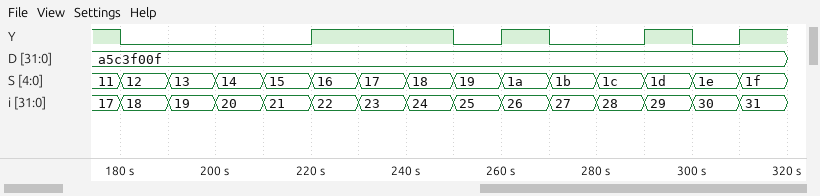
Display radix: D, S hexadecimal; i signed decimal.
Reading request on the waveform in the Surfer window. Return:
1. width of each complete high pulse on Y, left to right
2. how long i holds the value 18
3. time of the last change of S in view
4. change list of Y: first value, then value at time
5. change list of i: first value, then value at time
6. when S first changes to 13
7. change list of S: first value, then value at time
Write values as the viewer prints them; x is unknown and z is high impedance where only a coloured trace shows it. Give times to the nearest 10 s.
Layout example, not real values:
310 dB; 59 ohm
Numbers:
30 s, 10 s, 10 s; 10 s; 310 s; 1, 0 at 180 s, 1 at 220 s, 0 at 250 s, 1 at 260 s, 0 at 270 s, 1 at 290 s, 0 at 300 s, 1 at 310 s; 17, 18 at 180 s, 19 at 190 s, 20 at 200 s, 21 at 210 s, 22 at 220 s, 23 at 230 s, 24 at 240 s, 25 at 250 s, 26 at 260 s, 27 at 270 s, 28 at 280 s, 29 at 290 s, 30 at 300 s, 31 at 310 s; 190 s; 11, 12 at 180 s, 13 at 190 s, 14 at 200 s, 15 at 210 s, 16 at 220 s, 17 at 230 s, 18 at 240 s, 19 at 250 s, 1a at 260 s, 1b at 270 s, 1c at 280 s, 1d at 290 s, 1e at 300 s, 1f at 310 s
